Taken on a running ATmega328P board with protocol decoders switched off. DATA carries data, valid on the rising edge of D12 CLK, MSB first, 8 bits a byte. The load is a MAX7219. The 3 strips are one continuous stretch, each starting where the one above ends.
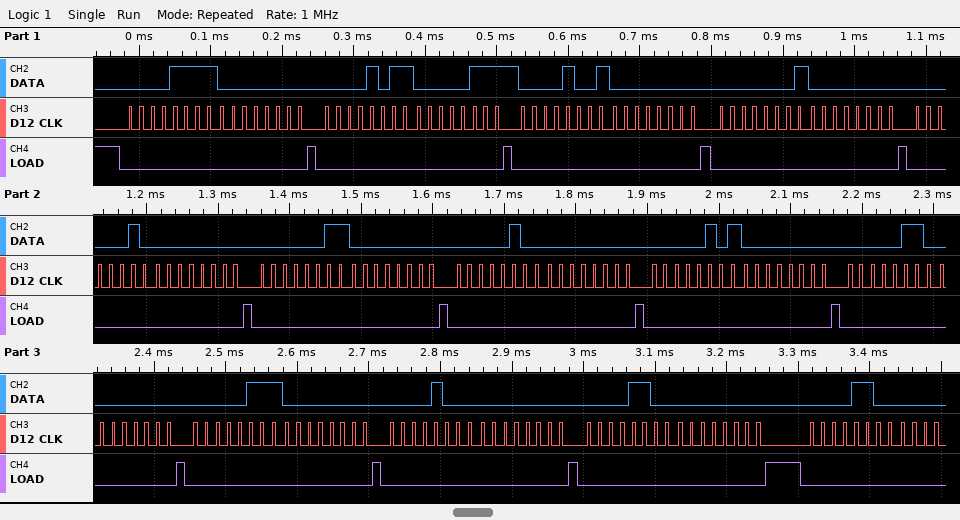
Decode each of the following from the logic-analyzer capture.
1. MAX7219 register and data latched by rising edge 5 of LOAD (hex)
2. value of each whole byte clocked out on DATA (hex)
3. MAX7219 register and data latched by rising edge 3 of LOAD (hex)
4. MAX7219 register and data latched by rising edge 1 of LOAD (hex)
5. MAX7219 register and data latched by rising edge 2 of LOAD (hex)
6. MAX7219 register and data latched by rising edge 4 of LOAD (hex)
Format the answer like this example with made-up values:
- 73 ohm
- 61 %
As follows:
- register 0x2, data 0x00
- 0F 00 0B 07 09 00 01 00 02 00 03 00 04 00 05 00 06 00 07 00 08 00 0C 00 0C
- register 0x9, data 0x00
- register 0xF, data 0x00
- register 0xB, data 0x07
- register 0x1, data 0x00
